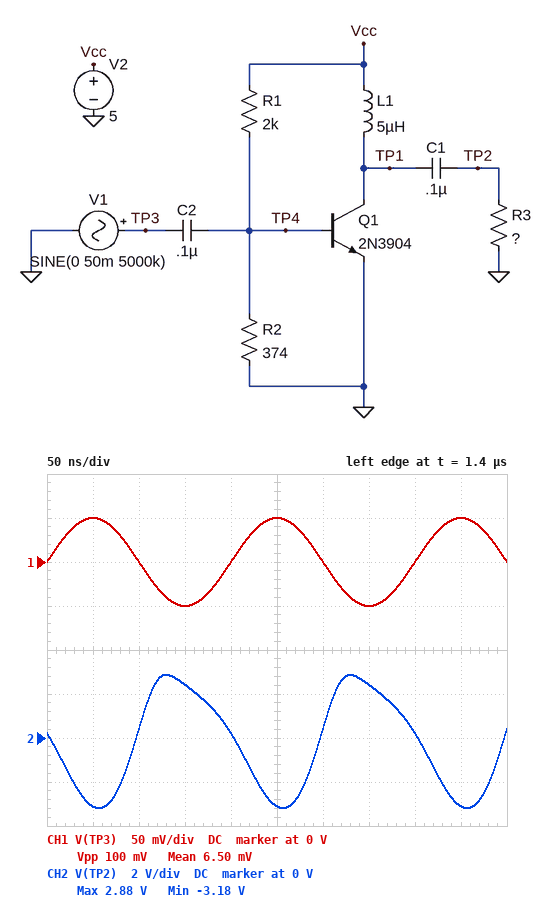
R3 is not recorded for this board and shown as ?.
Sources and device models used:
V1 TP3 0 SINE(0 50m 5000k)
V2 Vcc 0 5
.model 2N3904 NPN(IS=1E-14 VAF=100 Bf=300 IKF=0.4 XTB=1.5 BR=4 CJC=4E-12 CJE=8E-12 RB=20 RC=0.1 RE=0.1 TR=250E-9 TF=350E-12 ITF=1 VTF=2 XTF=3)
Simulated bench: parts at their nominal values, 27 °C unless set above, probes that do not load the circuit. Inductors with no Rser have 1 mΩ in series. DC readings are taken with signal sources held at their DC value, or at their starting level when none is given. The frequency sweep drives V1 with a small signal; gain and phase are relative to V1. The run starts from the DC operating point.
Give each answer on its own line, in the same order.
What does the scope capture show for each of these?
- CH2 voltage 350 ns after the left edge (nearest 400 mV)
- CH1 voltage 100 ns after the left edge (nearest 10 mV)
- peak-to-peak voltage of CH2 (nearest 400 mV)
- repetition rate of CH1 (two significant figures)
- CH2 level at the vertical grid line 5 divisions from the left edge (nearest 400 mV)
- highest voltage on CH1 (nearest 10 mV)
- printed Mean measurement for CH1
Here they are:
2.4 V
0 V
6.0 V
5.0 MHz
-3.2 V
50 mV
6.50 mV
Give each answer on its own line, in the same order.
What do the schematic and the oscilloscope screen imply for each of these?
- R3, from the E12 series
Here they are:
68 Ω
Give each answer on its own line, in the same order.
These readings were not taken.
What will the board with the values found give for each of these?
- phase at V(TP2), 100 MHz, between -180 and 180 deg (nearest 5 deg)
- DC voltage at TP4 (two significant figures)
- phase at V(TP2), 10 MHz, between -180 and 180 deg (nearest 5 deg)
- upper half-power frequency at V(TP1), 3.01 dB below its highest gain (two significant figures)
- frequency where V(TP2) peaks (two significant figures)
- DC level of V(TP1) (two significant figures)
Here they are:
95 deg
750 mV
160 deg
19 MHz
5.8 MHz
5.0 V
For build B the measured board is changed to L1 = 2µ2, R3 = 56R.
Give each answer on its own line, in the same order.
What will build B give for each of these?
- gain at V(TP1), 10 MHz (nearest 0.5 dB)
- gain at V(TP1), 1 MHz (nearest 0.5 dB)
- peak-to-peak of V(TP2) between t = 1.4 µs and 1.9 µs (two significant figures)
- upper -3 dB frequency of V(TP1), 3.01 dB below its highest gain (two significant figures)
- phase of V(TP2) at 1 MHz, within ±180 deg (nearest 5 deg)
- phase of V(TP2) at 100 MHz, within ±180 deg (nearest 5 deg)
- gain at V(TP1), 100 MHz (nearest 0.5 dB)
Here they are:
33.0 dB
22.5 dB
4.6 V
23 MHz
-105 deg
100 deg
19.0 dB
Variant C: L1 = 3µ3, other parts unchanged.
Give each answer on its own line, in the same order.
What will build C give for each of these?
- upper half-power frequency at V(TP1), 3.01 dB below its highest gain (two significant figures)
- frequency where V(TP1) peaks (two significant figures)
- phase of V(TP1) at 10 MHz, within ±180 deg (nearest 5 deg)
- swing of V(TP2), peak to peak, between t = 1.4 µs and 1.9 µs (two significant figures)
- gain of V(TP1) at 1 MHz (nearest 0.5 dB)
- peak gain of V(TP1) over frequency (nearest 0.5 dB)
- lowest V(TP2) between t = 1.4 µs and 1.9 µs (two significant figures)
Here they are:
21 MHz
7.2 MHz
165 deg
5.8 V
26.0 dB
35.0 dB
-2.9 V
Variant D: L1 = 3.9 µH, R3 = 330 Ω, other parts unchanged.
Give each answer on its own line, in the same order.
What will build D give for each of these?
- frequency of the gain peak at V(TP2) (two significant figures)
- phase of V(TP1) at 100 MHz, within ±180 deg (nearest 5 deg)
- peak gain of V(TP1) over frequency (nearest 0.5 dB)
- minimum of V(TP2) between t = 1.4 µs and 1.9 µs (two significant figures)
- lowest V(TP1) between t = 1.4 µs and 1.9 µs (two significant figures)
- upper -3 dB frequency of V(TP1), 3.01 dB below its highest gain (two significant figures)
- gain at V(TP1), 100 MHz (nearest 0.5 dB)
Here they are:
10 MHz
90 deg
45.5 dB
-4.8 V
230 mV
18 MHz
27.5 dB
